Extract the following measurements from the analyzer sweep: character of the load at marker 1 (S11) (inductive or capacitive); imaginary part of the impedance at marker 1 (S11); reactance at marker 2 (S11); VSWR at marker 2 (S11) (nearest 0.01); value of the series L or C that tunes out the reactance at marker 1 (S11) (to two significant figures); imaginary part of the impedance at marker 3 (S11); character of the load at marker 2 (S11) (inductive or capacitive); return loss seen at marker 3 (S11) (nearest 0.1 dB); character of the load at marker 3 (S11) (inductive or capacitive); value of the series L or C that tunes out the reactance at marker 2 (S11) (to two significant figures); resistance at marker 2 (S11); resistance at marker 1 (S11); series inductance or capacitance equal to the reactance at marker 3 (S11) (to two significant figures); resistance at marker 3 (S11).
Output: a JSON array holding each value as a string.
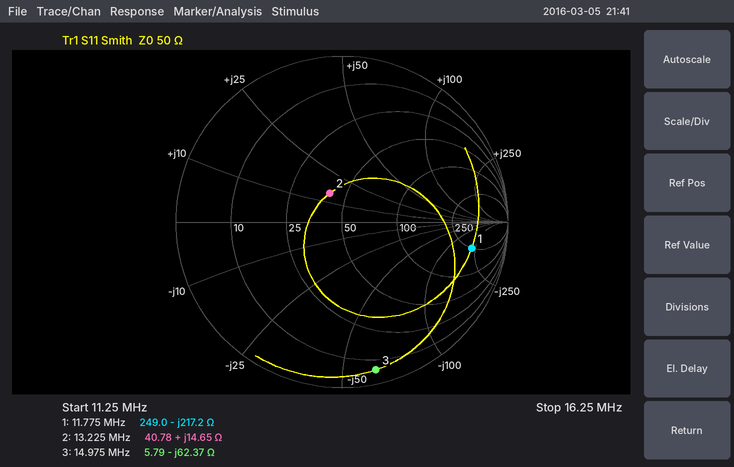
["capacitive", "-217.2 Ω", "+14.65 Ω", "1.46", "2.9 µH", "-62.37 Ω", "inductive", "0.8 dB", "capacitive", "820 pF", "40.78 Ω", "249.0 Ω", "170 pF", "5.79 Ω"]
